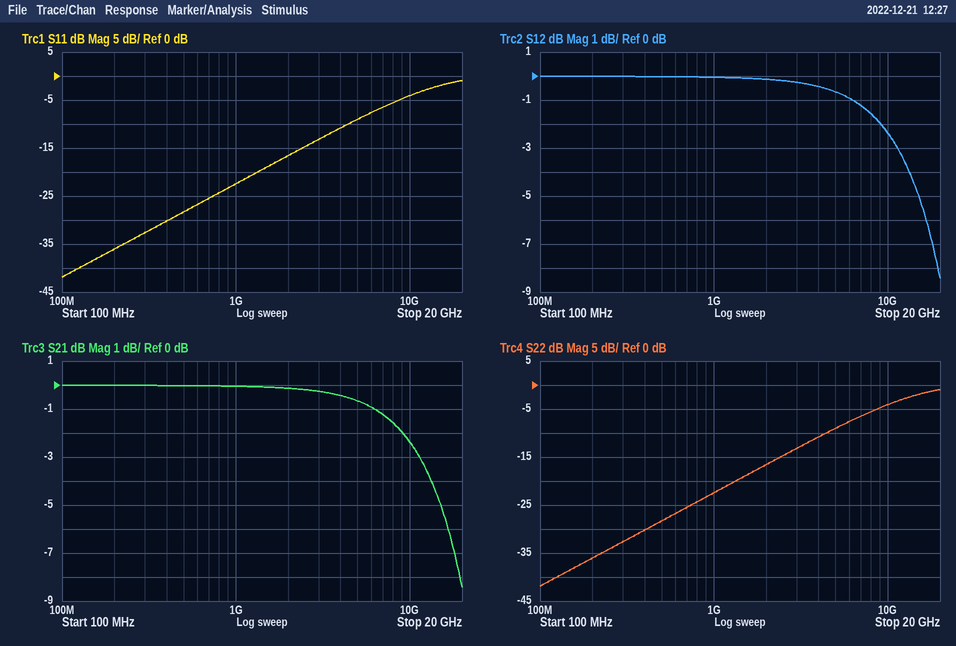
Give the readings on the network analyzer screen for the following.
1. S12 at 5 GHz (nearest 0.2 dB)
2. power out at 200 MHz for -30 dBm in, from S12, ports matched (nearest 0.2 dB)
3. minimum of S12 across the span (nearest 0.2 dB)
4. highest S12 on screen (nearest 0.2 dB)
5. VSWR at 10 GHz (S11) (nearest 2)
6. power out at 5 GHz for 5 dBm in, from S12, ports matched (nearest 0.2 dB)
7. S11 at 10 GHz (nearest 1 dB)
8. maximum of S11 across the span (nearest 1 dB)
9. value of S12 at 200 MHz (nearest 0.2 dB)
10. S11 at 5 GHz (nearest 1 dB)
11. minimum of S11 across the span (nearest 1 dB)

-0.6 dB
-30.0 dBm
-8.4 dB
0.0 dB
4
4.4 dBm
-4 dB
-1 dB
0.0 dB
-9 dB
-42 dB
